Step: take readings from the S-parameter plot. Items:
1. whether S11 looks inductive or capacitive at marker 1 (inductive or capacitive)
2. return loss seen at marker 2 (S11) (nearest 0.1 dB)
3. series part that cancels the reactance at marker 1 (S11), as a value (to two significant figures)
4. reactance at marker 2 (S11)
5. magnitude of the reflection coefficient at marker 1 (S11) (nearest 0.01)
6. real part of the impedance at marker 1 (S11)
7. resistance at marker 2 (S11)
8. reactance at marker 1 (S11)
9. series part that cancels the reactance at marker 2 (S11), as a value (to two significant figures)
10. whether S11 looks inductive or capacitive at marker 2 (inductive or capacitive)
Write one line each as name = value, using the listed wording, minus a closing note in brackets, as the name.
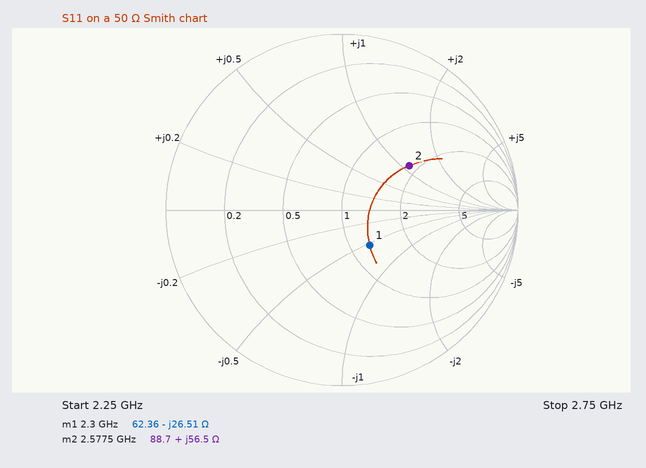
whether S11 looks inductive or capacitive at marker 1 = capacitive
return loss seen at marker 2 (S11) = 6.8 dB
series part that cancels the reactance at marker 1 (S11), as a value = 1.8 nH
reactance at marker 2 = +56.5 Ω
magnitude of the reflection coefficient at marker 1 (S11) = 0.25
real part of the impedance at marker 1 = 62.36 Ω
resistance at marker 2 = 88.7 Ω
reactance at marker 1 = -26.51 Ω
series part that cancels the reactance at marker 2 (S11), as a value = 1.1 pF
whether S11 looks inductive or capacitive at marker 2 = inductive
